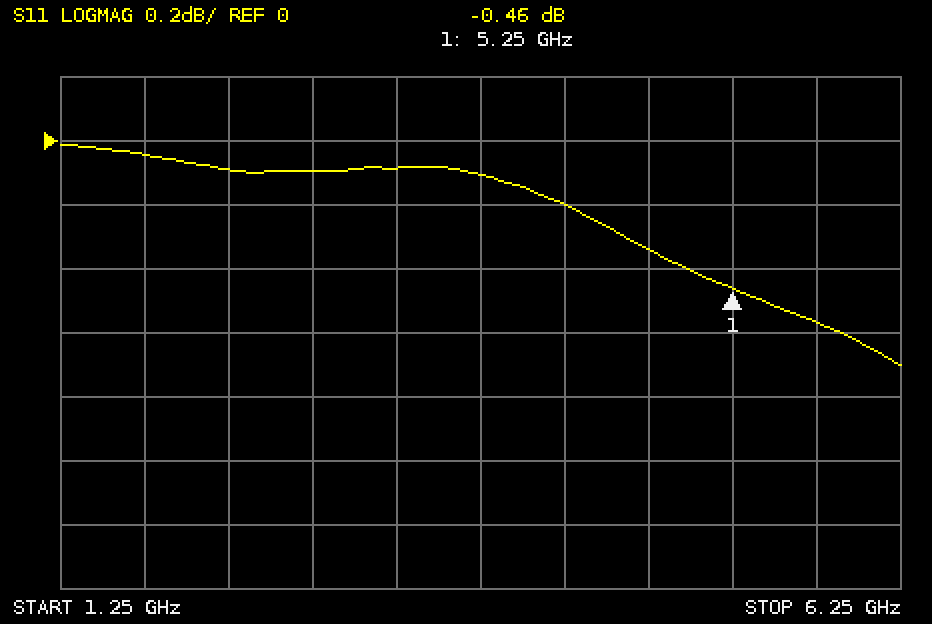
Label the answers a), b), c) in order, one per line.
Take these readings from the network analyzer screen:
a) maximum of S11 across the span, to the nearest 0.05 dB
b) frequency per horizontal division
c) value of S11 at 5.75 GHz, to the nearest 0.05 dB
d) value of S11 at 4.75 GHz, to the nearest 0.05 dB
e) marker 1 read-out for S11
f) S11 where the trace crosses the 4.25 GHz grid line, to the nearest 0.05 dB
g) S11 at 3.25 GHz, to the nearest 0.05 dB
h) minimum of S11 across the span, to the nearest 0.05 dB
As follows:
a) 0.00 dB
b) 500 MHz
c) -0.55 dB
d) -0.35 dB
e) -0.46 dB
f) -0.20 dB
g) -0.10 dB
h) -0.70 dB
